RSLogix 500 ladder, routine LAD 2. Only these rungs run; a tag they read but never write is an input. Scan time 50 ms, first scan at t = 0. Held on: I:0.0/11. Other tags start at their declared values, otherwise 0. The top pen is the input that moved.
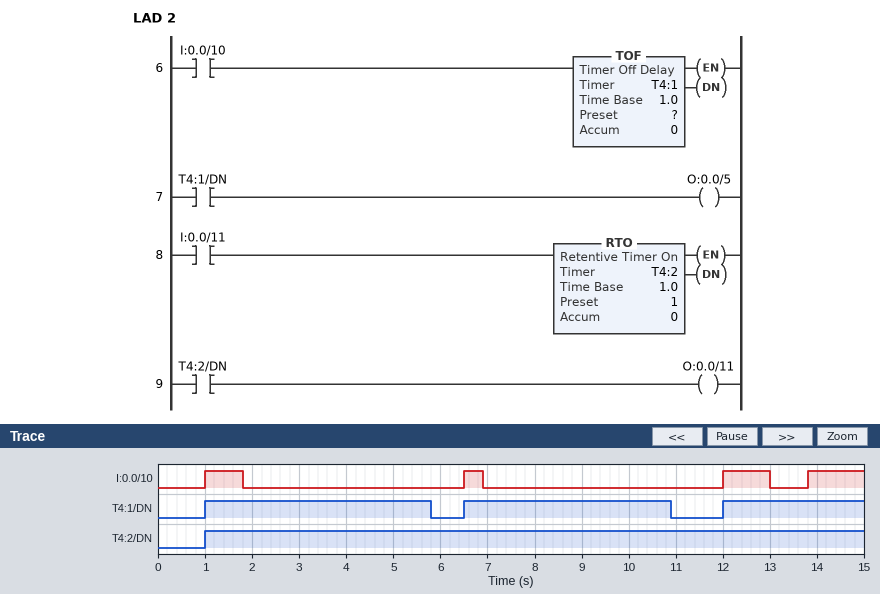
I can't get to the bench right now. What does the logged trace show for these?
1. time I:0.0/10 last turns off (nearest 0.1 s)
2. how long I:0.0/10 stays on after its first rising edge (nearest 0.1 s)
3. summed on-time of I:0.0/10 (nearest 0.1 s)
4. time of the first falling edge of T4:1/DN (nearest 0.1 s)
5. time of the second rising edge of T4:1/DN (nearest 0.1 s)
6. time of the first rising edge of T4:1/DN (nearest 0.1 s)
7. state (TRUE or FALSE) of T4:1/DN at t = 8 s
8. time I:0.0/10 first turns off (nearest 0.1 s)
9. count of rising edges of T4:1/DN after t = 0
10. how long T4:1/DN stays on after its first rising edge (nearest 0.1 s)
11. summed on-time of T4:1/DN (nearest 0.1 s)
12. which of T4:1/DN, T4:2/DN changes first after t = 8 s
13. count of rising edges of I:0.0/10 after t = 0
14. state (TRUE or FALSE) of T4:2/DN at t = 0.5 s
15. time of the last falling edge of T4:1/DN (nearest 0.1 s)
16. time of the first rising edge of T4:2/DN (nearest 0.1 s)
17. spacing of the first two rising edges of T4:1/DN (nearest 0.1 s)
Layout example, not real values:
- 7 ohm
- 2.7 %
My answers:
- 13.0 s
- 0.8 s
- 3.4 s
- 5.8 s
- 6.5 s
- 1.0 s
- TRUE
- 1.8 s
- 3
- 4.8 s
- 12.2 s
- T4:1/DN
- 4
- FALSE
- 10.9 s
- 1.0 s
- 5.5 s
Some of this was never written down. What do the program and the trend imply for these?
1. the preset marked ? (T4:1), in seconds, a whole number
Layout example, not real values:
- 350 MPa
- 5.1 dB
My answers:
- 4 s
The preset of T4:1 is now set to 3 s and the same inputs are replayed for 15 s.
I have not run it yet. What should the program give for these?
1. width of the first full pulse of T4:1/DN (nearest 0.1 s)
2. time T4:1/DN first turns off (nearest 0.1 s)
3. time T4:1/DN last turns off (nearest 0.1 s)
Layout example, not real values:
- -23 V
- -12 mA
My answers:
- 3.8 s
- 4.8 s
- 9.9 s
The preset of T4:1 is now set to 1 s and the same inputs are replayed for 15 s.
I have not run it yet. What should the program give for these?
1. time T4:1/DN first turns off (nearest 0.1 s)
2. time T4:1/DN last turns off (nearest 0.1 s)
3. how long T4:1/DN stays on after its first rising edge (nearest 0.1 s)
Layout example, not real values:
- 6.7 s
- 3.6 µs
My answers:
- 2.8 s
- 7.9 s
- 1.8 s
